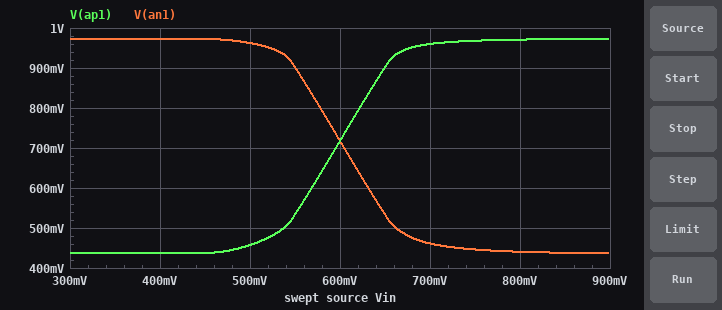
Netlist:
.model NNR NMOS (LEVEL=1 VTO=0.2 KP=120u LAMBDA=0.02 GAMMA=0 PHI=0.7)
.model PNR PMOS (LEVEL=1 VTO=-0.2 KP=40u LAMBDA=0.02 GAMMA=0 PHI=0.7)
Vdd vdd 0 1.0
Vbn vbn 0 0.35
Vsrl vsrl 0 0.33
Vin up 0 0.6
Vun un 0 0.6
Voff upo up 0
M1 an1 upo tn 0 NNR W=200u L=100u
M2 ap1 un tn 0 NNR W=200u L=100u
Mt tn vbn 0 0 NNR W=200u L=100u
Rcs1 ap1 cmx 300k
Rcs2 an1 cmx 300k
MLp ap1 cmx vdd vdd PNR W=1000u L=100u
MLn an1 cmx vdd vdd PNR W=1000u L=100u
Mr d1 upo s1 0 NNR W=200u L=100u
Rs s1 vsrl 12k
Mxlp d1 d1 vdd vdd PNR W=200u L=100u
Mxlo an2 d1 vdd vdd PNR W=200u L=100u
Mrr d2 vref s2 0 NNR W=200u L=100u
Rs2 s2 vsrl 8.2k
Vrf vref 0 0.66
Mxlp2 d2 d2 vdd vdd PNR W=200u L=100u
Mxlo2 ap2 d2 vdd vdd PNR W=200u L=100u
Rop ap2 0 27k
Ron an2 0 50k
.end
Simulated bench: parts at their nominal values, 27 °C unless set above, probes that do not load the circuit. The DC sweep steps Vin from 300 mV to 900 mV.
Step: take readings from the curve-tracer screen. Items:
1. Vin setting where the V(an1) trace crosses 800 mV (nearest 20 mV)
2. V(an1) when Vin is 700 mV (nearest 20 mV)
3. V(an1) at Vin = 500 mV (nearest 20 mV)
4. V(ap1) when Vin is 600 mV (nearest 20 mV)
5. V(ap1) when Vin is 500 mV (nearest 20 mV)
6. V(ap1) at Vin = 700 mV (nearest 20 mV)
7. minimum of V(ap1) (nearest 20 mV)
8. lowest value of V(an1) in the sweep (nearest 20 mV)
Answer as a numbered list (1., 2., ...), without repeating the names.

1. 580 mV
2. 460 mV
3. 960 mV
4. 720 mV
5. 460 mV
6. 960 mV
7. 440 mV
8. 440 mV
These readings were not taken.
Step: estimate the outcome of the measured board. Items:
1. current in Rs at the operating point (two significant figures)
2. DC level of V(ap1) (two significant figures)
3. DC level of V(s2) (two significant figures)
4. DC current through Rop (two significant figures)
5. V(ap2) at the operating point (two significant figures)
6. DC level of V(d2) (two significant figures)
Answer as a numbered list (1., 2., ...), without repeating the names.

1. 500 nA
2. 720 mV
3. 340 mV
4. 1.7 µA
5. 45 mV
6. 600 mV
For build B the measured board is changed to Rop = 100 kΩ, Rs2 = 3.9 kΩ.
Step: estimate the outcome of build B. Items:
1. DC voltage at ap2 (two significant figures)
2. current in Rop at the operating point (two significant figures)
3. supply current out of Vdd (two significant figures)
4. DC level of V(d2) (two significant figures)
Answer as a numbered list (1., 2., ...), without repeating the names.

1. 180 mV
2. 1.8 µA
3. 7.4 µA
4. 590 mV
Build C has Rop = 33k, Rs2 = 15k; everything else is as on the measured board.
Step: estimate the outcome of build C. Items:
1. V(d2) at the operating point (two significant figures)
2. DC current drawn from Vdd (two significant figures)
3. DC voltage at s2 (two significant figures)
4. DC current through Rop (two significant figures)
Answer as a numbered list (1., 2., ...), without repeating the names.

1. 610 mV
2. 6.6 µA
3. 350 mV
4. 1.4 µA
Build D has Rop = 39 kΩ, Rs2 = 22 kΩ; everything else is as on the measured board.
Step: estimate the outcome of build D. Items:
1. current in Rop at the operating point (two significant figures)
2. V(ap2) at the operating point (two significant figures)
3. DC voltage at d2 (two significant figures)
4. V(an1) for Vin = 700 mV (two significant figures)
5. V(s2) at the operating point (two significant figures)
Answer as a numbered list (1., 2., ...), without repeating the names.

1. 1.3 µA
2. 50 mV
3. 620 mV
4. 460 mV
5. 360 mV
